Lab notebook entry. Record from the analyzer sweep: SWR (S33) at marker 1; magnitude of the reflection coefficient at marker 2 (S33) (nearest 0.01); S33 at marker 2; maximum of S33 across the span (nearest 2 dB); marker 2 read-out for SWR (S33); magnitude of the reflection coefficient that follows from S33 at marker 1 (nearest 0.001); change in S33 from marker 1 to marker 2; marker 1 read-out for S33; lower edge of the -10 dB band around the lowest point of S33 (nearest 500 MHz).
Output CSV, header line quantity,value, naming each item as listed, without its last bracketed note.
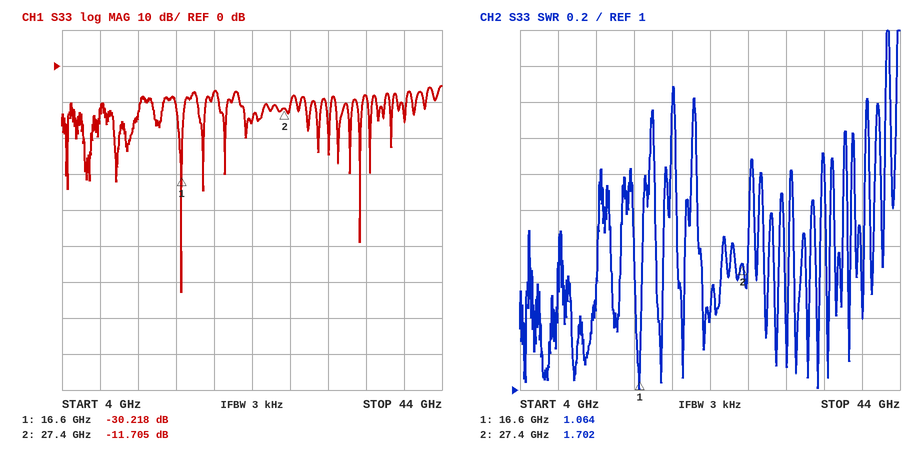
quantity,value
SWR (S33) at marker 1,1.064
magnitude of the reflection coefficient at marker 2 (S33),0.26
S33 at marker 2,-11.705 dB
maximum of S33 across the span,-6 dB
marker 2 read-out for SWR,1.702
magnitude of the reflection coefficient that follows from S33 at marker 1,0.031
change in S33 from marker 1 to marker 2,18.513 dB
marker 1 read-out for S33,-30.218 dB
lower edge of the -10 dB band around the lowest point of S33,16.0 GHz
